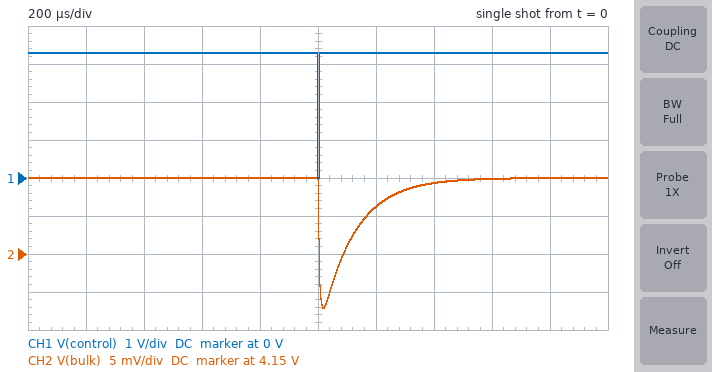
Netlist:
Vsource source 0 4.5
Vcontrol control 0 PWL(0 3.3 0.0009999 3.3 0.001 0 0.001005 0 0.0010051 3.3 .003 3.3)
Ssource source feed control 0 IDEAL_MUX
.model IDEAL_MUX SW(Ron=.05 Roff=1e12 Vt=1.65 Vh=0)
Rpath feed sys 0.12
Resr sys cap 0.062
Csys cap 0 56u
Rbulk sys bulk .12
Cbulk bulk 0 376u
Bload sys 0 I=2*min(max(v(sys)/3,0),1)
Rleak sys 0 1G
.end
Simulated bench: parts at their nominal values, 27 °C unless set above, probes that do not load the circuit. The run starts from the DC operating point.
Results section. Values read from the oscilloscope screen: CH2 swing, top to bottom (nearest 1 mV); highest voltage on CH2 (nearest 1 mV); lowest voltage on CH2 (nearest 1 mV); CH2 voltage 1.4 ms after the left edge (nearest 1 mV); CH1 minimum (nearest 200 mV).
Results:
17 mV
4.160 V
4.143 V
4.159 V
0 V
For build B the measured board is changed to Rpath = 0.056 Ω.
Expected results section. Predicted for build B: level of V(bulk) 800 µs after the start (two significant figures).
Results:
4.3 V
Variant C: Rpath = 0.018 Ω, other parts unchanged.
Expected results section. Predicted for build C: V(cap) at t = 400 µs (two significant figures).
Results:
4.4 V
